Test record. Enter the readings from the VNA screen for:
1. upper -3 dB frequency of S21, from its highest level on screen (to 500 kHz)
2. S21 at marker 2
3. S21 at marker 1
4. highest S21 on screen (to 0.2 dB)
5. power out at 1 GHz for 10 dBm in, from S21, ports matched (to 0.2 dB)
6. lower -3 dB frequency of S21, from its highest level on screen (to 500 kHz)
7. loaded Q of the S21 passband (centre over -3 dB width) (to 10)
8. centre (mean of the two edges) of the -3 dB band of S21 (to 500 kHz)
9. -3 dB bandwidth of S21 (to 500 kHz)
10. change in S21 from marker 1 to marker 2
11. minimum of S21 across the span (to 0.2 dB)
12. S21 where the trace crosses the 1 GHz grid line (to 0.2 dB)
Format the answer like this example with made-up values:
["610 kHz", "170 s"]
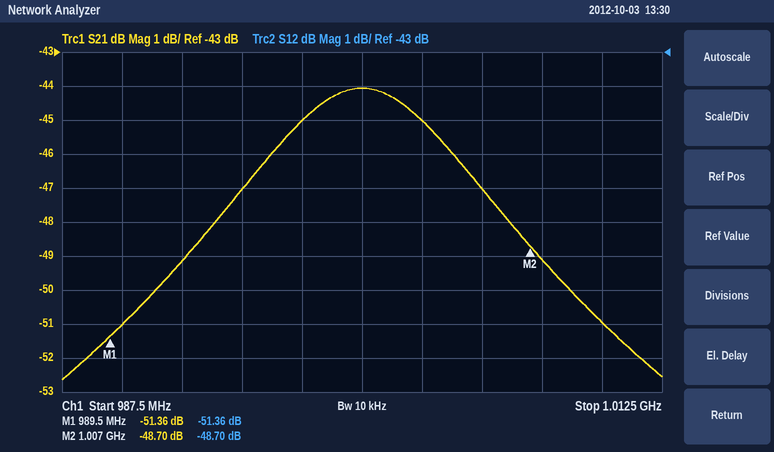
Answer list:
["1.0050 GHz", "-48.70 dB", "-51.36 dB", "-44.0 dB", "-34.0 dBm", "995.0 MHz", "100", "1.0000 GHz", "10.0 MHz", "2.66 dB", "-52.6 dB", "-44.0 dB"]
